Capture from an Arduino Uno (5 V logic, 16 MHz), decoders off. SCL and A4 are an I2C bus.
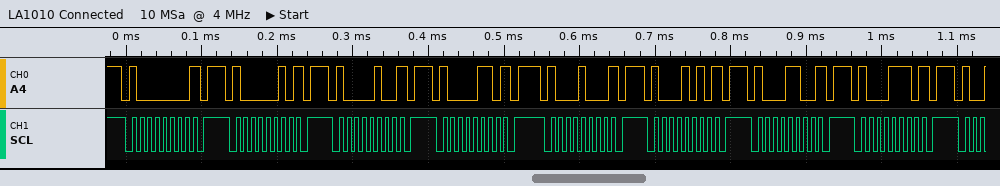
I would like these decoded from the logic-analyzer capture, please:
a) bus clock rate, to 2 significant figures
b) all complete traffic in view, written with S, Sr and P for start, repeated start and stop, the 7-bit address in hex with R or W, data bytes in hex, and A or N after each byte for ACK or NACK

100 kHz
S 40W N P S 41W N P S 42W N P S 43W N P S 44W N P S 45W N P S 46W N P S 47W N P
